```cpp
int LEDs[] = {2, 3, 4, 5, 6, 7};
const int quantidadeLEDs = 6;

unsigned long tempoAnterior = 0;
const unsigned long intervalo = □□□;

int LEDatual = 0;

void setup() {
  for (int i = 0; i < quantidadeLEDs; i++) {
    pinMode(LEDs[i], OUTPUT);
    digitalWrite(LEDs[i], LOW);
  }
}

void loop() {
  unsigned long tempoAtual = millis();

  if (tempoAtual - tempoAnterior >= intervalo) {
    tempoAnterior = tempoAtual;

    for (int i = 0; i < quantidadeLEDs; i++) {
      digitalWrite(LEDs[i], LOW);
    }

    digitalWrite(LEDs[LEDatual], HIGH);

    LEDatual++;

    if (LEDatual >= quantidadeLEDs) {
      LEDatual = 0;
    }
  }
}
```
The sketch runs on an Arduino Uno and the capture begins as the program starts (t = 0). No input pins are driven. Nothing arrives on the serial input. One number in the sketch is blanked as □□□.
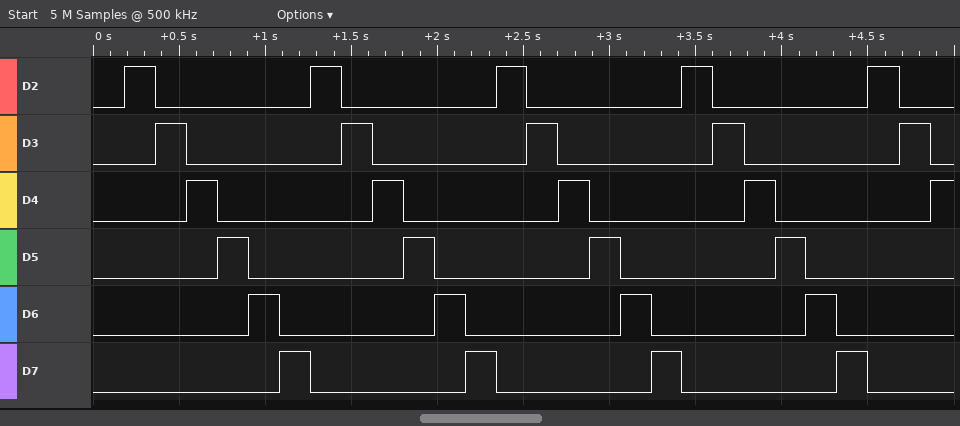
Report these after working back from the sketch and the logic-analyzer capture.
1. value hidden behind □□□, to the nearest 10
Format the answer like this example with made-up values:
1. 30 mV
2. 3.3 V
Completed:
1. 180
